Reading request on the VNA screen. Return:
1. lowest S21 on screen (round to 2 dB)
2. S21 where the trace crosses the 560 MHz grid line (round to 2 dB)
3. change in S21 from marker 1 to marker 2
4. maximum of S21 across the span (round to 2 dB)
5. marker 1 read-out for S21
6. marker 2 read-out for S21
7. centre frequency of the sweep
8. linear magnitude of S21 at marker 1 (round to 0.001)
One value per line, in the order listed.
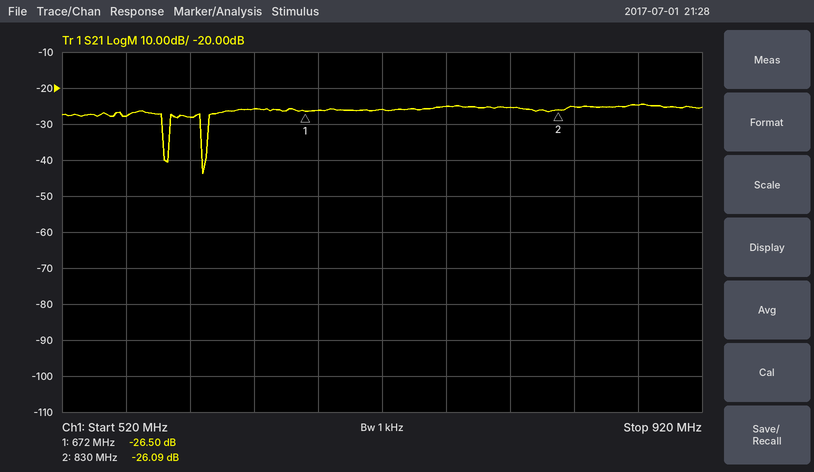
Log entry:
-44 dB
-28 dB
0.41 dB
-24 dB
-26.50 dB
-26.09 dB
720 MHz
0.047
